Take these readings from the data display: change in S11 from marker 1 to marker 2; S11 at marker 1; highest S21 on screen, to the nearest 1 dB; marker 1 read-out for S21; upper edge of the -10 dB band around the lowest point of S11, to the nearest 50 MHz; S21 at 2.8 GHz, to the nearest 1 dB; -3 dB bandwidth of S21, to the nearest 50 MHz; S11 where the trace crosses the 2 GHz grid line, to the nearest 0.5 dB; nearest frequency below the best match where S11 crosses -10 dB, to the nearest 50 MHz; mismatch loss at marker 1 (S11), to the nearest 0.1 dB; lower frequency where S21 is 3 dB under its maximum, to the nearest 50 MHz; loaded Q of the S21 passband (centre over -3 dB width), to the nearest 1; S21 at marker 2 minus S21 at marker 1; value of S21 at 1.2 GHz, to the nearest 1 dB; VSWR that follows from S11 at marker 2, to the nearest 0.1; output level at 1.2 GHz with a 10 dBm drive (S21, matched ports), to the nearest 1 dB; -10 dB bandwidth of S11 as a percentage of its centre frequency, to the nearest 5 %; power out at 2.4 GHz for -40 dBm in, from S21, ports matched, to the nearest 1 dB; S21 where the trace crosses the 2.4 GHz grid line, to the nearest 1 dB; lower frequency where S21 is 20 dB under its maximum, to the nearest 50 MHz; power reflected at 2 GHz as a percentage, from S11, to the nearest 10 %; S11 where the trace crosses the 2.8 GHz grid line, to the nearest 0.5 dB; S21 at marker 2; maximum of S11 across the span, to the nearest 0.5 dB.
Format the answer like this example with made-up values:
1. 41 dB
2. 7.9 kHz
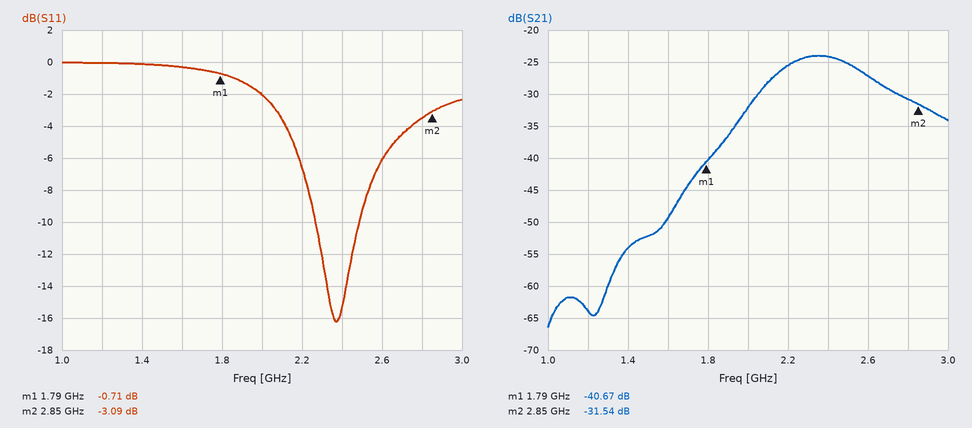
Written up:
1. -2.38 dB
2. -0.71 dB
3. -24 dB
4. -40.67 dB
5. 2.50 GHz
6. -31 dB
7. 450 MHz
8. -2.0 dB
9. 2.25 GHz
10. 8.2 dB
11. 2.15 GHz
12. 5
13. 9.13 dB
14. -64 dB
15. 5.7
16. -54 dBm
17. 10 %
18. -64 dBm
19. -24 dB
20. 1.70 GHz
21. 60 %
22. -3.5 dB
23. -31.54 dB
24. 0.0 dB
